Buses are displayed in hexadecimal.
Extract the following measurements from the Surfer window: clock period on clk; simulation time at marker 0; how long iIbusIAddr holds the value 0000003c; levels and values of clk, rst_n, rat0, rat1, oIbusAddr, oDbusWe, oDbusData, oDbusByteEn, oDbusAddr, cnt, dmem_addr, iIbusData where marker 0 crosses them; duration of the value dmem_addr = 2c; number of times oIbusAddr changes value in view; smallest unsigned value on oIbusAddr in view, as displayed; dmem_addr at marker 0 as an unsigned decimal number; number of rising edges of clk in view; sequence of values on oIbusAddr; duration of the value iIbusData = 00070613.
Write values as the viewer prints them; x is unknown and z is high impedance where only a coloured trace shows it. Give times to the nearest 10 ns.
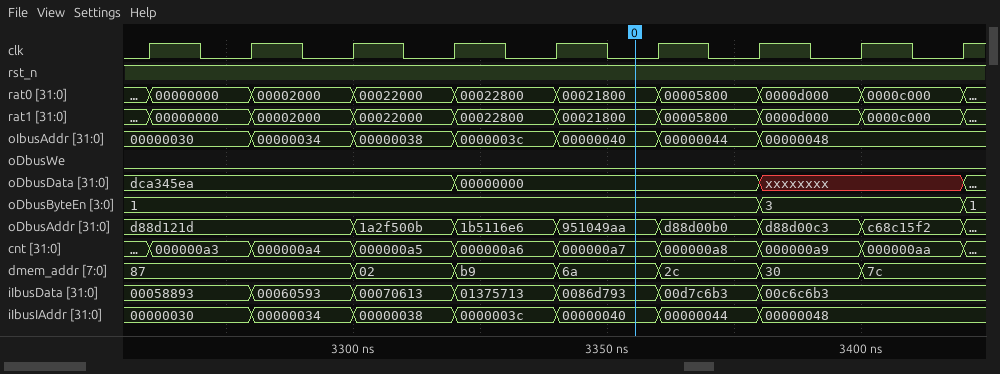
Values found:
20 ns
3360 ns
20 ns
clk=0, rst_n=1, rat0=00021800, rat1=00021800, oIbusAddr=00000040, oDbusWe=0, oDbusData=00000000, oDbusByteEn=1, oDbusAddr=951049aa, cnt=000000a7, dmem_addr=6a, iIbusData=0086d793
20 ns
6
00000030
106
9
00000030, 00000034, 00000038, 0000003c, 00000040, 00000044, 00000048
20 ns
